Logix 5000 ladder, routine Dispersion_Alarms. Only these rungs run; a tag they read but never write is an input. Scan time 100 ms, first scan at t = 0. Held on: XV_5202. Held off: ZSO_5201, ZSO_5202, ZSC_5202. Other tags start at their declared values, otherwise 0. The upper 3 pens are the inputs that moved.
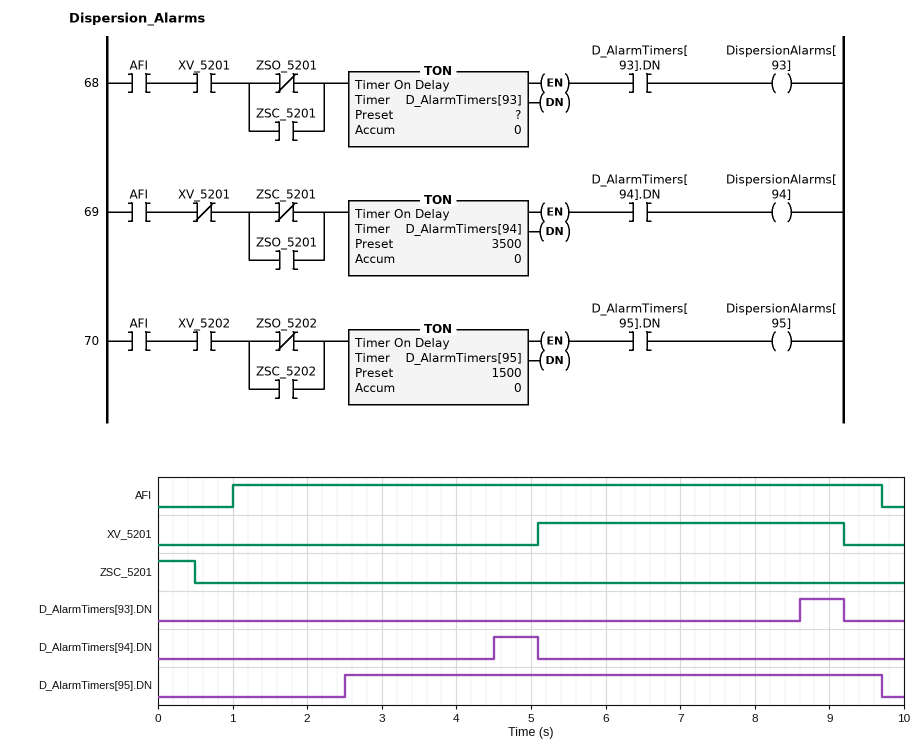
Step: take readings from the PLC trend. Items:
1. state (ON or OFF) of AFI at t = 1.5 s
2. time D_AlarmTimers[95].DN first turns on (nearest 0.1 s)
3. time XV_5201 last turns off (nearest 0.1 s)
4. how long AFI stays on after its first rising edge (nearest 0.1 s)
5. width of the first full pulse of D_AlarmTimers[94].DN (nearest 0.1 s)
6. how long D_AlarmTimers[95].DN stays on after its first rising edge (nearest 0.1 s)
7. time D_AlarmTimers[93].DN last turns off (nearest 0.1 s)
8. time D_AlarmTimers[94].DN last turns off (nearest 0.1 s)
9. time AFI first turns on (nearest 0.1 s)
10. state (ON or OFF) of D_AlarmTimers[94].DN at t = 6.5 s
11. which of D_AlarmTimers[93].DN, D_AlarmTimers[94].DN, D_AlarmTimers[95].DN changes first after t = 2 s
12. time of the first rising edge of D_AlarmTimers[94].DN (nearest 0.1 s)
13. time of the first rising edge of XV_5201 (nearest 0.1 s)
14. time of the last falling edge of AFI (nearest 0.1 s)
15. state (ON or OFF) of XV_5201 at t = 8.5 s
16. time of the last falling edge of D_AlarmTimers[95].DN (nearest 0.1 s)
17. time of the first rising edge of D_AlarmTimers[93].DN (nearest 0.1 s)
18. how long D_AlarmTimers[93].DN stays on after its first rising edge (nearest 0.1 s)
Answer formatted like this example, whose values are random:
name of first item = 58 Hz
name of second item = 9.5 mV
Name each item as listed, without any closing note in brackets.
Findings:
state (ON or OFF) of AFI at t = 1.5 s = ON
time D_AlarmTimers[95].DN first turns on = 2.5 s
time XV_5201 last turns off = 9.2 s
how long AFI stays on after its first rising edge = 8.7 s
width of the first full pulse of D_AlarmTimers[94].DN = 0.6 s
how long D_AlarmTimers[95].DN stays on after its first rising edge = 7.2 s
time D_AlarmTimers[93].DN last turns off = 9.2 s
time D_AlarmTimers[94].DN last turns off = 5.1 s
time AFI first turns on = 1.0 s
state (ON or OFF) of D_AlarmTimers[94].DN at t = 6.5 s = OFF
which of D_AlarmTimers[93].DN, D_AlarmTimers[94].DN, D_AlarmTimers[95].DN changes first after t = 2 s = D_AlarmTimers[95].DN
time of the first rising edge of D_AlarmTimers[94].DN = 4.5 s
time of the first rising edge of XV_5201 = 5.1 s
time of the last falling edge of AFI = 9.7 s
state (ON or OFF) of XV_5201 at t = 8.5 s = ON
time of the last falling edge of D_AlarmTimers[95].DN = 9.7 s
time of the first rising edge of D_AlarmTimers[93].DN = 8.6 s
how long D_AlarmTimers[93].DN stays on after its first rising edge = 0.6 s
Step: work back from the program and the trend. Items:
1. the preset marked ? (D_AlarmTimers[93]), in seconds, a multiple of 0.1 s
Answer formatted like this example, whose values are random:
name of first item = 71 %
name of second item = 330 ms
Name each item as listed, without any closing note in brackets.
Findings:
the preset marked ? (D_AlarmTimers[93]), in seconds, a multiple of 0.1 s = 3.5 s
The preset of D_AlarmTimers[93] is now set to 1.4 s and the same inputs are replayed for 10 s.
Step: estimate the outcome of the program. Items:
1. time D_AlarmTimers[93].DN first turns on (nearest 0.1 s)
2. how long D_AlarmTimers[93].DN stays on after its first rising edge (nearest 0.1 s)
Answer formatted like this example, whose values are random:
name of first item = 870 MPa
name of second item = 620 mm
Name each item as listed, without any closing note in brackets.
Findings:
time D_AlarmTimers[93].DN first turns on = 6.5 s
how long D_AlarmTimers[93].DN stays on after its first rising edge = 2.7 s
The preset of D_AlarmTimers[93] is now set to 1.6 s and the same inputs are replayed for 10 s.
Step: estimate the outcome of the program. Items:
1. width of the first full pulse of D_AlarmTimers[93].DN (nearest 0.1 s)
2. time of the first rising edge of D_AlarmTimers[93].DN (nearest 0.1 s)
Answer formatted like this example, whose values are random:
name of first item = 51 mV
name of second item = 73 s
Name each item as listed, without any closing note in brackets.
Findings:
width of the first full pulse of D_AlarmTimers[93].DN = 2.5 s
time of the first rising edge of D_AlarmTimers[93].DN = 6.7 s
